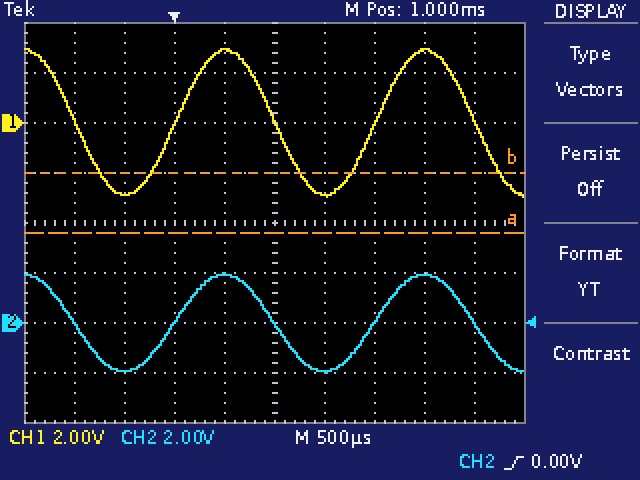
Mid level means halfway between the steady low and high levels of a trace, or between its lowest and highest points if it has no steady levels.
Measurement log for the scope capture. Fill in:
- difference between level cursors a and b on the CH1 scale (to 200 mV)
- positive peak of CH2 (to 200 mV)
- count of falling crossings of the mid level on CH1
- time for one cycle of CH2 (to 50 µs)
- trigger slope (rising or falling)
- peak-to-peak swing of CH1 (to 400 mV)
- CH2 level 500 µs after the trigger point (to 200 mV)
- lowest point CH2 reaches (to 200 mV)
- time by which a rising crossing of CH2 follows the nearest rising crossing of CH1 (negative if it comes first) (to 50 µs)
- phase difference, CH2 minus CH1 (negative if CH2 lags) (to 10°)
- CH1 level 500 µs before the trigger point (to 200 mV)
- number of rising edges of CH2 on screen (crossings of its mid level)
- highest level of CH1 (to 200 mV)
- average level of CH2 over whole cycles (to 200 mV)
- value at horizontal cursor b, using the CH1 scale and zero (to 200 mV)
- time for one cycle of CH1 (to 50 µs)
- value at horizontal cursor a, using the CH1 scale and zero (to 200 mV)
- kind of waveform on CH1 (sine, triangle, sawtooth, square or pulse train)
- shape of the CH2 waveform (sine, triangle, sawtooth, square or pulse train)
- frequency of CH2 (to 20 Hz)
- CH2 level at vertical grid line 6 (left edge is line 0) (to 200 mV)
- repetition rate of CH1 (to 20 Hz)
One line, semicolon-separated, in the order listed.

2.4 V; 2.0 V; 3; 2.00 ms; rising; 6.0 V; 2.0 V; -2.0 V; 0 µs; 0°; -2.8 V; 2; 3.0 V; 0.0 V; -2.0 V; 2.00 ms; -4.4 V; sine; sine; 500 Hz; -2.0 V; 500 Hz
